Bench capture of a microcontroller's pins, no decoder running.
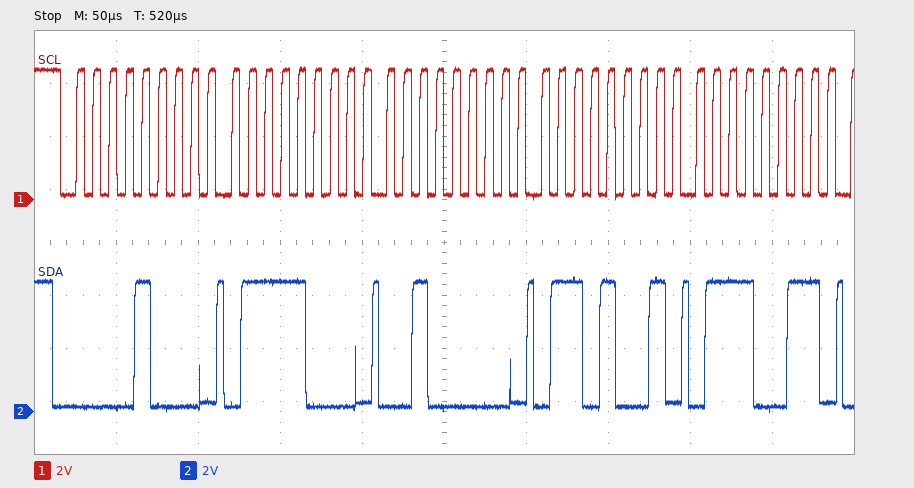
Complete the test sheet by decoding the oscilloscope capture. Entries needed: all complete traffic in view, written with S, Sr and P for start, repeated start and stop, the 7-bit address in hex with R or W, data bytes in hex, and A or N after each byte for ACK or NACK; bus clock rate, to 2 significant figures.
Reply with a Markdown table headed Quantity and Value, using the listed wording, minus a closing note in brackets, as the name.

| Quantity | Value |
|---|---|
| all complete traffic in view, written with S, Sr and P for start, repeated start and stop, the 7-bit address in hex with R or W, data bytes in hex, and A or N after each byte for ACK or NACK | S 04W A 78 A 20 A 69 A 73 A |
| bus clock rate, to 2 significant figures | 100 kHz |
